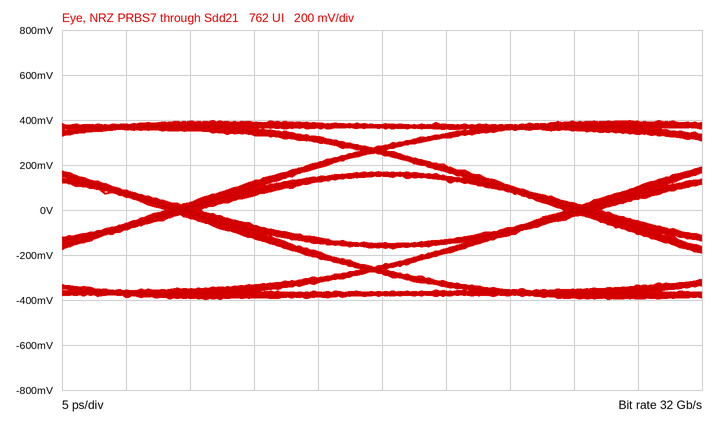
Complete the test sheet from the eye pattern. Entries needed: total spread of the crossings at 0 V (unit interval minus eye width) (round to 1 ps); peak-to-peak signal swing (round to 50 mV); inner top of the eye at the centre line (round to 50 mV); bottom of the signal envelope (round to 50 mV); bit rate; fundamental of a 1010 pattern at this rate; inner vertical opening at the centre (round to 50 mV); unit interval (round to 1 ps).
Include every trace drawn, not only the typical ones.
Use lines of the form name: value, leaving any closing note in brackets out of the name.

total spread of the crossings at 0 V (unit interval minus eye width): 3 ps
peak-to-peak signal swing: 800 mV
inner top of the eye at the centre line: 150 mV
bottom of the signal envelope: -400 mV
bit rate: 32 Gb/s
fundamental of a 1010 pattern at this rate: 16 GHz
inner vertical opening at the centre: 300 mV
unit interval: 31 ps
